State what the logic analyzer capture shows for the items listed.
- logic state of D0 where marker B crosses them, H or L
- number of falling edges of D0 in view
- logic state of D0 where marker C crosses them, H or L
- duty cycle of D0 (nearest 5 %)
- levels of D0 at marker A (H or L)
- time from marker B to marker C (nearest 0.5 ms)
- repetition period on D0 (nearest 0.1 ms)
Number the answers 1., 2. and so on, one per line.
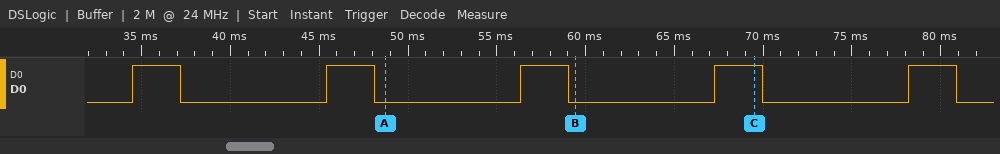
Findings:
1. D0=L
2. 5
3. D0=H
4. 25 %
5. D0=L
6. 10 ms
7. 10.9 ms
